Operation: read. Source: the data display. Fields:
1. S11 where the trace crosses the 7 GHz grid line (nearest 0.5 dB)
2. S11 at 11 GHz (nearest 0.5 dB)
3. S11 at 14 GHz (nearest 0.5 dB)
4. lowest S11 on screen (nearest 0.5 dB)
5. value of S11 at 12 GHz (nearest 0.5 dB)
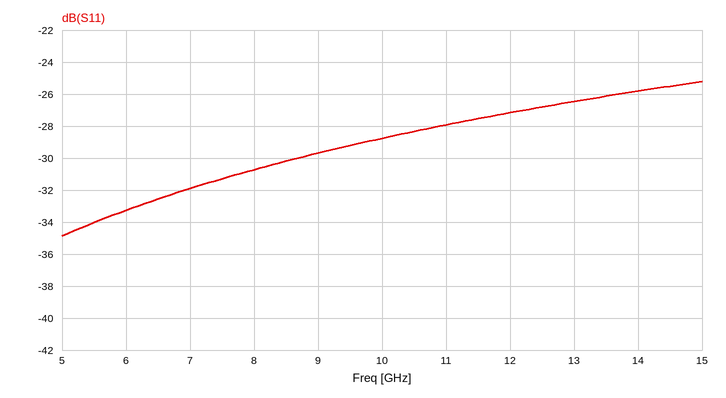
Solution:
-32.0 dB
-28.0 dB
-26.0 dB
-35.0 dB
-27.0 dB
